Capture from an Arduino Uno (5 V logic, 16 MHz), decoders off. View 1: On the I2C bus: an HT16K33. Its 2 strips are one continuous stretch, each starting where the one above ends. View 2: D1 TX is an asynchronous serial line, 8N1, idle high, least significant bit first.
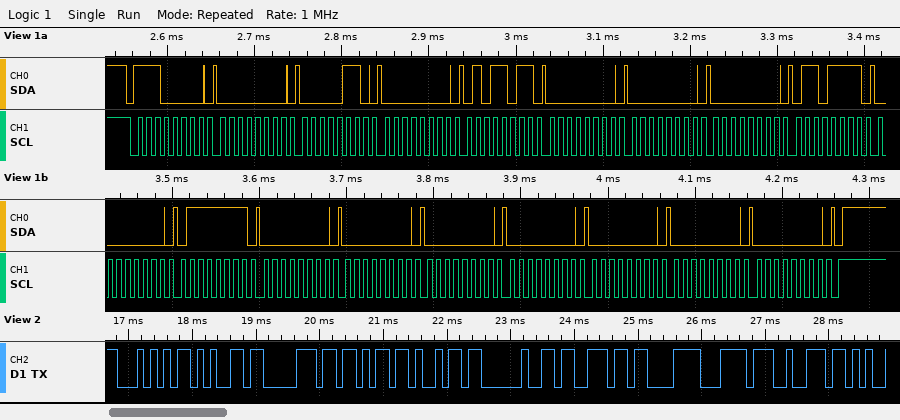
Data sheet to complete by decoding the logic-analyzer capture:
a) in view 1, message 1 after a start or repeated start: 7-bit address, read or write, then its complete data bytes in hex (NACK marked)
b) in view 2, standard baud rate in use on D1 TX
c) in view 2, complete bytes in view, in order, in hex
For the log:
0x70 write: 00 06 00 5B 00 00 00 6F 00 7F 00 00 00 00 00 00 00
9600 baud
54 65 70 6B 69 20 73 C3 BC 72
